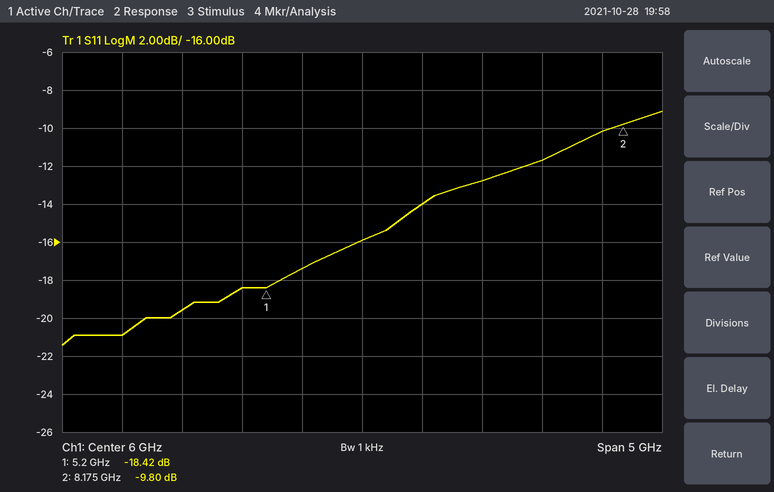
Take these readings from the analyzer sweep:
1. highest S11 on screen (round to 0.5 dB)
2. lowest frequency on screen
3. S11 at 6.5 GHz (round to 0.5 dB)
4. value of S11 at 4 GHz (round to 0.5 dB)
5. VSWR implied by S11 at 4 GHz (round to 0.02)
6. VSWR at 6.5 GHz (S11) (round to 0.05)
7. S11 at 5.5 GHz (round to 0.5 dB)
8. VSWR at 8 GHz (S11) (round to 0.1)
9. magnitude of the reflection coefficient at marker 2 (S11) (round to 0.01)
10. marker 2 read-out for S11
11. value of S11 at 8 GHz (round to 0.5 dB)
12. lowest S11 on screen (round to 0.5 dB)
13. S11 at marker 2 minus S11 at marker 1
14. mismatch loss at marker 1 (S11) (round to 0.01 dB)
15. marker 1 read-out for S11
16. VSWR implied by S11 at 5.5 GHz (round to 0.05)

-9.0 dB
3.5 GHz
-14.0 dB
-21.0 dB
1.20
1.50
-17.5 dB
1.9
0.32
-9.80 dB
-10.0 dB
-21.5 dB
8.62 dB
0.06 dB
-18.42 dB
1.30
